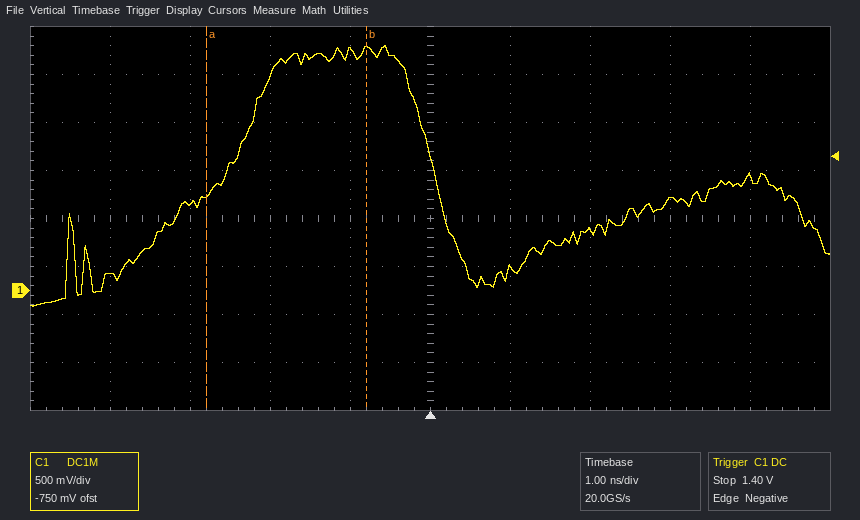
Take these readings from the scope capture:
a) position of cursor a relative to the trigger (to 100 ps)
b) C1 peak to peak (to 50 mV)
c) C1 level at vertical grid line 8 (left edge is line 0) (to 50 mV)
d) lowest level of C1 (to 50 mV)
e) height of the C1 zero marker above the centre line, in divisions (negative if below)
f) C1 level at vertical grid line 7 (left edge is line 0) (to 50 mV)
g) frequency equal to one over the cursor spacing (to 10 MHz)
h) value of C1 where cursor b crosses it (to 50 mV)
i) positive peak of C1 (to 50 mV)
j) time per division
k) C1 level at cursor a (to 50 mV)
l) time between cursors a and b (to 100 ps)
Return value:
-2.8 ns
2.70 V
950 mV
-150 mV
-1.5 div
600 mV
500 MHz
2.50 V
2.55 V
1 ns
1.00 V
2.0 ns
